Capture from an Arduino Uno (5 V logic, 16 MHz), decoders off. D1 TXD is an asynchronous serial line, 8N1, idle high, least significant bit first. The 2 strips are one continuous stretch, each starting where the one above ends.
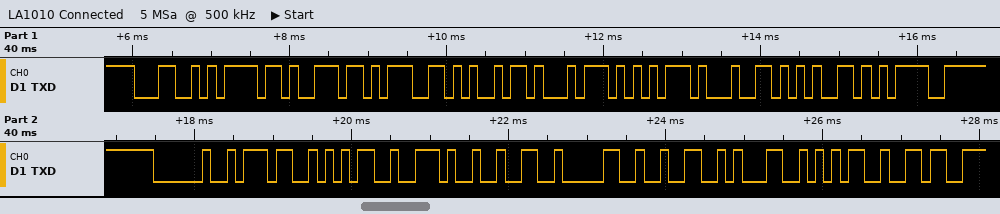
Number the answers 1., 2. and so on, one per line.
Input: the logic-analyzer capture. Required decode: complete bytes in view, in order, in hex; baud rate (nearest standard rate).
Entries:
1. 0x4C 0x6F 0x6E 0x67 0x69 0x74 0x75 0x64 0x65 0x3D 0x20 0x37 0x35 0x2E 0x32 0x30 0x32 0x31 0x35 0x36
2. 9600 baud
